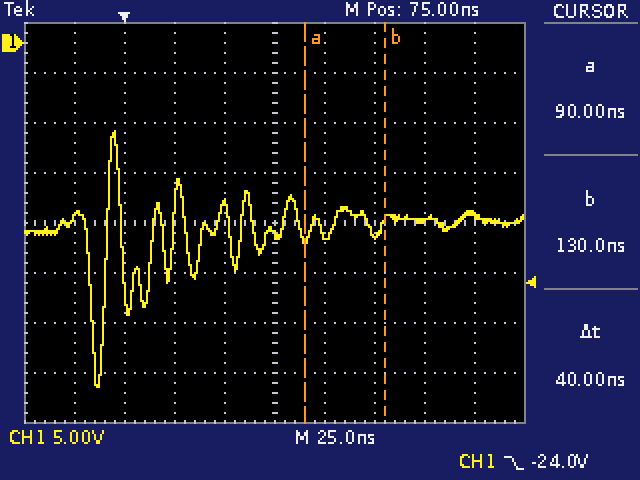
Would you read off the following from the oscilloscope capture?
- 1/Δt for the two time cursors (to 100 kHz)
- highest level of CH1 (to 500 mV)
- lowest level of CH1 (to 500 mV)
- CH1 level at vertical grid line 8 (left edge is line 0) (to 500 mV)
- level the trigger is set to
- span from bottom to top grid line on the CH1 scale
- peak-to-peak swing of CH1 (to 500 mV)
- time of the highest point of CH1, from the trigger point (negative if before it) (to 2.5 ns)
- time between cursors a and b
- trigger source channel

25.0 MHz
-9.0 V
-34.5 V
-18.0 V
-24.0 V
40 V
25.5 V
-5.0 ns
40 ns
CH1
